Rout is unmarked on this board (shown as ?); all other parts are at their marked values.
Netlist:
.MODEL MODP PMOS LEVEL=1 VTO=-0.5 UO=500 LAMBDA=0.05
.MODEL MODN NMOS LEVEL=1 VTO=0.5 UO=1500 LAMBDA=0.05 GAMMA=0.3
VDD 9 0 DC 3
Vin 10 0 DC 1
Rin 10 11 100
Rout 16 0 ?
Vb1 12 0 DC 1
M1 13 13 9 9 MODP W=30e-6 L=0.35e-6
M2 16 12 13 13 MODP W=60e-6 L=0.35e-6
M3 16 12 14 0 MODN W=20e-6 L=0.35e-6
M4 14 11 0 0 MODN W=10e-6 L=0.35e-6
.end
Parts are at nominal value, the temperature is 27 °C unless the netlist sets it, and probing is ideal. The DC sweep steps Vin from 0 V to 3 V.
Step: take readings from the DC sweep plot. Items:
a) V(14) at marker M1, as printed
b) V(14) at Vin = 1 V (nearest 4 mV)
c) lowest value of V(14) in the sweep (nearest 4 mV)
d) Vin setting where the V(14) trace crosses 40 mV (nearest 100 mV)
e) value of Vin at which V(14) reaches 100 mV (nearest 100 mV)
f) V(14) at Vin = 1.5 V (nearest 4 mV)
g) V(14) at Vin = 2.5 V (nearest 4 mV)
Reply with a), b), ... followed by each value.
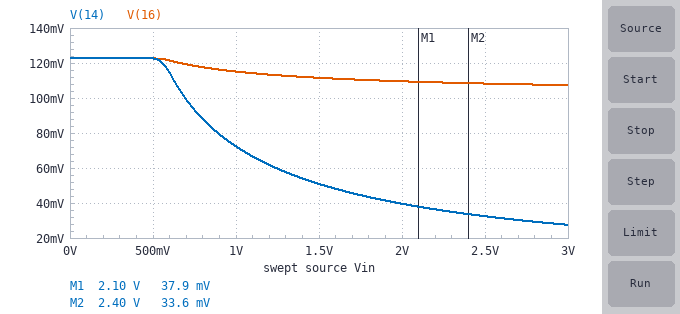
a) 37.9 mV
b) 72 mV
c) 28 mV
d) 2.0 V
e) 700 mV
f) 52 mV
g) 32 mV
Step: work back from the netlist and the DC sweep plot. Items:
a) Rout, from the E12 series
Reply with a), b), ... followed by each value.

a) 390 Ω
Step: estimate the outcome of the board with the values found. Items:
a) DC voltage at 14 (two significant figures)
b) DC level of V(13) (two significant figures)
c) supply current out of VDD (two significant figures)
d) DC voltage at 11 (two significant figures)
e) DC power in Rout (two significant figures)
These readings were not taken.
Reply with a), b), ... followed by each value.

a) 72 mV
b) 1.9 V
c) 310 µA
d) 1.0 V
e) 34 µW
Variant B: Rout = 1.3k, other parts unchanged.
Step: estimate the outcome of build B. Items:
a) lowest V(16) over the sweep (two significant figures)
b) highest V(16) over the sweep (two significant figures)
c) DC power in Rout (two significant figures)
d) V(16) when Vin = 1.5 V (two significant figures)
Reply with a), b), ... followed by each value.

a) 300 mV
b) 410 mV
c) 96 µW
d) 330 mV
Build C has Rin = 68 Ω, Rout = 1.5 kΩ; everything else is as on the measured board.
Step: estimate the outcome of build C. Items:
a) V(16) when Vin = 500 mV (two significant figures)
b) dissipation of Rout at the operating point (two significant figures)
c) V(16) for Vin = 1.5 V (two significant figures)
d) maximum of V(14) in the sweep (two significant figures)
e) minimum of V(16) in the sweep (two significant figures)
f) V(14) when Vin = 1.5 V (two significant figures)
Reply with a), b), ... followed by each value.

a) 470 mV
b) 110 µW
c) 370 mV
d) 430 mV
e) 330 mV
f) 120 mV
